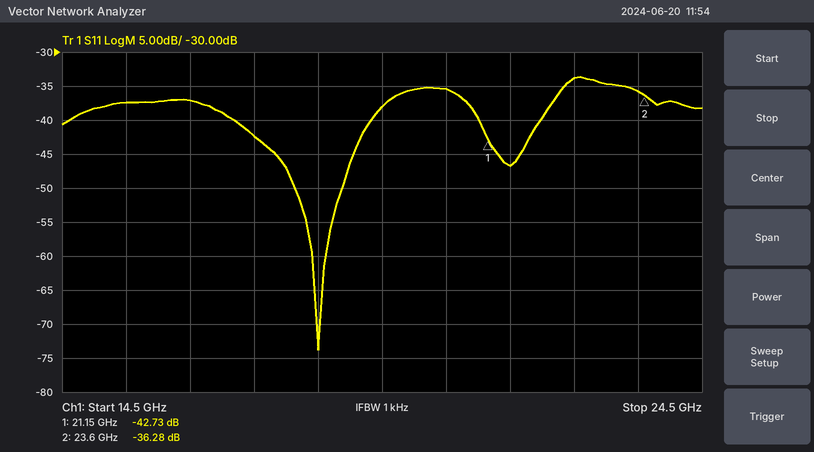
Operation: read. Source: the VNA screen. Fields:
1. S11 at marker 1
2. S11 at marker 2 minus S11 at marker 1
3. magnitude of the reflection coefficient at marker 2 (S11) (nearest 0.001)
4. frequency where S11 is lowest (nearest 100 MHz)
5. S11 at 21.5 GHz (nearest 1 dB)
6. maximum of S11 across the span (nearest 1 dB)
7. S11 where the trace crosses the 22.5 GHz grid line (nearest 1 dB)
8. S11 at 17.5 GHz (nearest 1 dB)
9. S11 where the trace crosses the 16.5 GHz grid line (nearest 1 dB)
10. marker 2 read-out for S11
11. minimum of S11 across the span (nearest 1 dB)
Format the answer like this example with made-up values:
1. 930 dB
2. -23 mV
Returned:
1. -42.73 dB
2. 6.45 dB
3. 0.015
4. 18.5 GHz
5. -47 dB
6. -34 dB
7. -34 dB
8. -42 dB
9. -37 dB
10. -36.28 dB
11. -74 dB
